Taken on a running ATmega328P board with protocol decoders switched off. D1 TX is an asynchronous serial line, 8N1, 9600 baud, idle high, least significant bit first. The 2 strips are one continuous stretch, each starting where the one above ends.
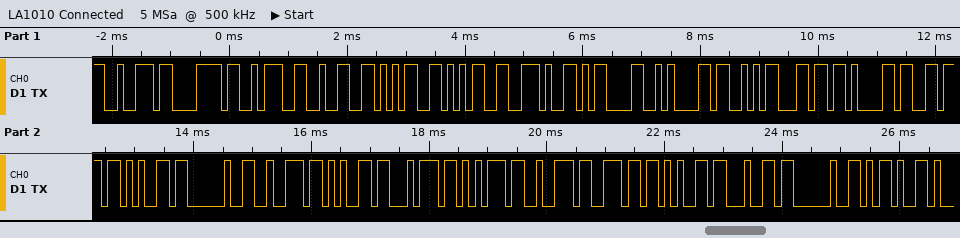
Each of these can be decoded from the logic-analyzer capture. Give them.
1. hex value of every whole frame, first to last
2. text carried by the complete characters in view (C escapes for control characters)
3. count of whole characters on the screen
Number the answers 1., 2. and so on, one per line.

1. 72 78 3A 32 35 35 2E 0D 0A 53 6C 61 76 65 20 72 65 74 75 72 6E 65 64 20 2D
2. "rx:255.\r\nSlave returned -"
3. 25
